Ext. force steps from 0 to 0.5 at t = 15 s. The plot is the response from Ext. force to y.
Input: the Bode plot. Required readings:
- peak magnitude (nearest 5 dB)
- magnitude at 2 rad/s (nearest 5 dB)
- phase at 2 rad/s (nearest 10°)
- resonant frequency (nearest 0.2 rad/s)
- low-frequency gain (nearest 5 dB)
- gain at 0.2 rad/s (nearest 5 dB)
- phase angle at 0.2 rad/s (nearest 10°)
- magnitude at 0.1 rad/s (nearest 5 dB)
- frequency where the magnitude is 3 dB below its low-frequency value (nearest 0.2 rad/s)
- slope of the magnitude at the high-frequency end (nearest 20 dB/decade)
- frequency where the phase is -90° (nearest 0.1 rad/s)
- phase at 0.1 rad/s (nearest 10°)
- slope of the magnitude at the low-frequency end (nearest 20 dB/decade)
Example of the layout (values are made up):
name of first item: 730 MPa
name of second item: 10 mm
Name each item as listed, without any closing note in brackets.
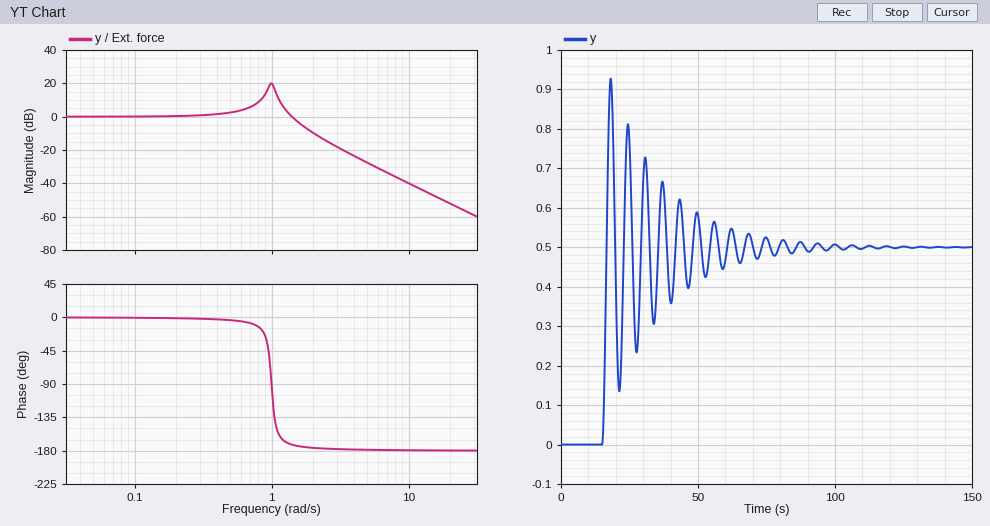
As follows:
peak magnitude: 20 dB
magnitude at 2 rad/s: -10 dB
phase at 2 rad/s: -180°
resonant frequency: 1.0 rad/s
low-frequency gain: 0 dB
gain at 0.2 rad/s: 0 dB
phase angle at 0.2 rad/s: 0°
magnitude at 0.1 rad/s: 0 dB
frequency where the magnitude is 3 dB below its low-frequency value: 1.6 rad/s
slope of the magnitude at the high-frequency end: -40 dB/decade
frequency where the phase is -90°: 1.0 rad/s
phase at 0.1 rad/s: 0°
slope of the magnitude at the low-frequency end: 0 dB/decade
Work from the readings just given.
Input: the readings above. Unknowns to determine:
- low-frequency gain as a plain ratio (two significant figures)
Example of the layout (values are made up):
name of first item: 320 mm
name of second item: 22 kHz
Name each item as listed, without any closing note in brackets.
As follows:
low-frequency gain as a plain ratio: 1.0
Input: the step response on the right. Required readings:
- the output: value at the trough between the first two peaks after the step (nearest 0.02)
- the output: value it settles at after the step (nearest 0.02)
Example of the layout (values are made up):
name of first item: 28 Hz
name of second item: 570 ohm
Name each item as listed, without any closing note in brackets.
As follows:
the output: value at the trough between the first two peaks after the step: 0.14
the output: value it settles at after the step: 0.50
